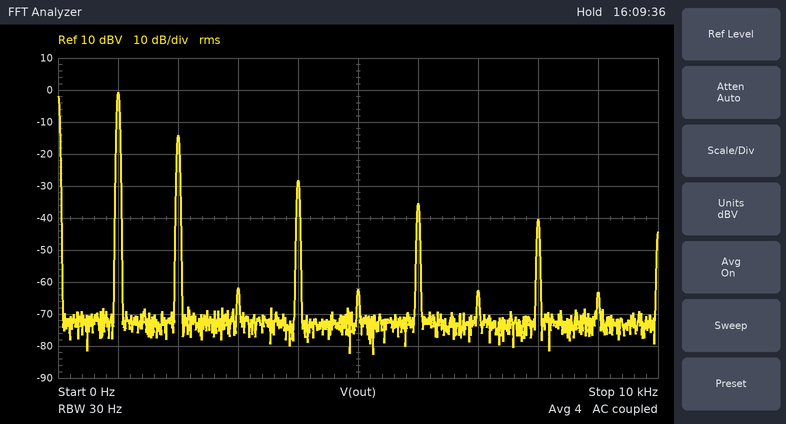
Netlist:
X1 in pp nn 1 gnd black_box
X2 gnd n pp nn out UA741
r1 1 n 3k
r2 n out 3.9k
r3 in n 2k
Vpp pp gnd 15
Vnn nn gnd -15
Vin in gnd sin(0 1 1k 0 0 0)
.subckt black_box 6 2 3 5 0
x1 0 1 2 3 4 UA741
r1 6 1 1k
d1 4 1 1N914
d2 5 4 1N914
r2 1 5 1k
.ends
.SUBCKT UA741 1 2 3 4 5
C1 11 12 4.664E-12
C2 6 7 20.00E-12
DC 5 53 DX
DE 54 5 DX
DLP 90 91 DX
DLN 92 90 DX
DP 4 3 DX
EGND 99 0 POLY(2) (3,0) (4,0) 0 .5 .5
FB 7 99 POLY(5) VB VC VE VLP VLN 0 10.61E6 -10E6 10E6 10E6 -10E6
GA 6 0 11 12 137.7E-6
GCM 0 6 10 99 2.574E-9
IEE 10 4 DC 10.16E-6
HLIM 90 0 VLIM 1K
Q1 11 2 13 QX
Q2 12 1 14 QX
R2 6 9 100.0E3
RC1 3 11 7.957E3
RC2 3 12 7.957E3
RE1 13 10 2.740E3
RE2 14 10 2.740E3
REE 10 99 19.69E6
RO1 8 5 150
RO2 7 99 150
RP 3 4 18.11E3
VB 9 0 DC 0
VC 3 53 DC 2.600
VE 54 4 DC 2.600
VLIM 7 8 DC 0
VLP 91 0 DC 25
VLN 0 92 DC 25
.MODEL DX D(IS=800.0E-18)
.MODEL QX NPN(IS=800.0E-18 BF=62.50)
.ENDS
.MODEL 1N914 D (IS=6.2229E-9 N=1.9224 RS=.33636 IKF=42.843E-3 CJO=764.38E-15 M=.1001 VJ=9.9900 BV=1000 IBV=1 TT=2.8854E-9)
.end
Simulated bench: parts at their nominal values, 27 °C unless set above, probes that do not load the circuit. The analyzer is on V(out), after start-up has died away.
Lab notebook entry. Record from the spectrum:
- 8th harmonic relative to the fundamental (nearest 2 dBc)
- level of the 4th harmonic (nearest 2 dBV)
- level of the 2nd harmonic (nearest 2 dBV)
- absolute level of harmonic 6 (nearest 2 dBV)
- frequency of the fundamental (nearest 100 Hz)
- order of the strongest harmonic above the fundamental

-40 dBc
-28 dBV
-14 dBV
-36 dBV
1.0 kHz
2
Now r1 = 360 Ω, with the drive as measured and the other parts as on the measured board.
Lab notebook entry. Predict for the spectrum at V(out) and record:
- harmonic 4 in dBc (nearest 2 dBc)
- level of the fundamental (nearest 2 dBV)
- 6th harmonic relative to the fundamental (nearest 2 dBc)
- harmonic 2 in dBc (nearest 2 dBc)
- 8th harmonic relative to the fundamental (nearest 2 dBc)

-18 dBc
8 dBV
-24 dBc
-4 dBc
-30 dBc
